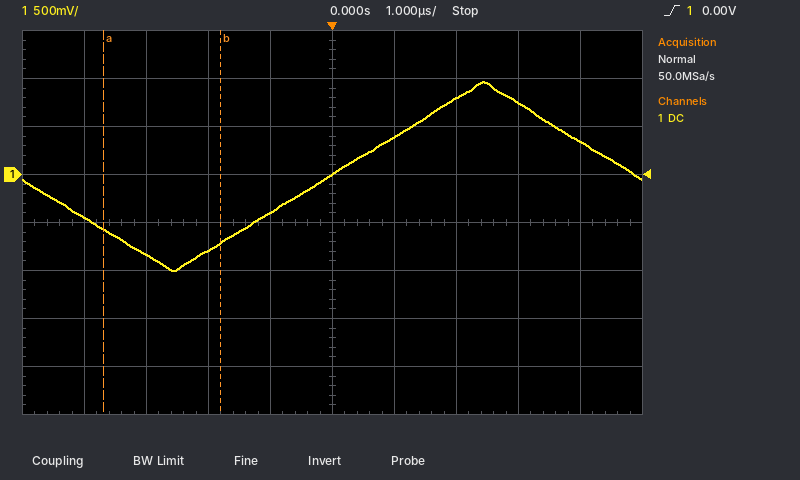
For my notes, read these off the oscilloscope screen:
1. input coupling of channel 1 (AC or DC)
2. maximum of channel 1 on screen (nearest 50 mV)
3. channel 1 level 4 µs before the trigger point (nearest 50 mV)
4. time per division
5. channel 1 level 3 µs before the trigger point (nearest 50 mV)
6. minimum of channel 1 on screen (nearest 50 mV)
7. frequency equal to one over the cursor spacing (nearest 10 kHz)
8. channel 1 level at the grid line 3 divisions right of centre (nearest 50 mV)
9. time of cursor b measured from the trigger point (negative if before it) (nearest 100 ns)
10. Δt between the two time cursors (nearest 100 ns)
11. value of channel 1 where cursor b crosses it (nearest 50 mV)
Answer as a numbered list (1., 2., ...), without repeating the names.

1. DC
2. 950 mV
3. -450 mV
4. 1 µs
5. -850 mV
6. -1.00 V
7. 530 kHz
8. 750 mV
9. -1.8 µs
10. 1.9 µs
11. -700 mV
